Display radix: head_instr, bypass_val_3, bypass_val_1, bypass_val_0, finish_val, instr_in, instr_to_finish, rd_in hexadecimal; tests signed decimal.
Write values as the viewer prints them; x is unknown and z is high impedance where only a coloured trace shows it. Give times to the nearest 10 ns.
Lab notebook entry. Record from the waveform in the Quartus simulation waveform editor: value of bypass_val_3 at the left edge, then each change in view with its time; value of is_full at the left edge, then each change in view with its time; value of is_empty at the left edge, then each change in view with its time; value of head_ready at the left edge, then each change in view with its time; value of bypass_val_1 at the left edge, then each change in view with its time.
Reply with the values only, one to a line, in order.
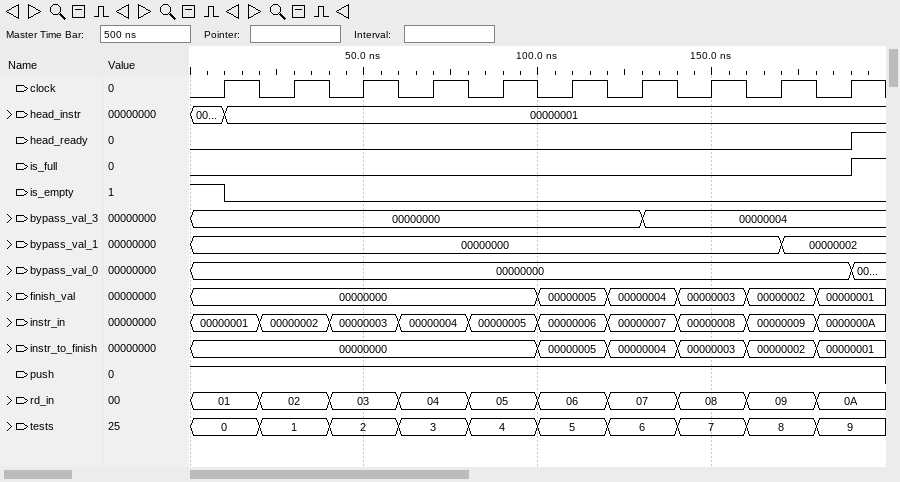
00000000, 00000004 at 130 ns
0, 1 at 190 ns
1, 0 at 10 ns
0, 1 at 190 ns
00000000, 00000002 at 170 ns
